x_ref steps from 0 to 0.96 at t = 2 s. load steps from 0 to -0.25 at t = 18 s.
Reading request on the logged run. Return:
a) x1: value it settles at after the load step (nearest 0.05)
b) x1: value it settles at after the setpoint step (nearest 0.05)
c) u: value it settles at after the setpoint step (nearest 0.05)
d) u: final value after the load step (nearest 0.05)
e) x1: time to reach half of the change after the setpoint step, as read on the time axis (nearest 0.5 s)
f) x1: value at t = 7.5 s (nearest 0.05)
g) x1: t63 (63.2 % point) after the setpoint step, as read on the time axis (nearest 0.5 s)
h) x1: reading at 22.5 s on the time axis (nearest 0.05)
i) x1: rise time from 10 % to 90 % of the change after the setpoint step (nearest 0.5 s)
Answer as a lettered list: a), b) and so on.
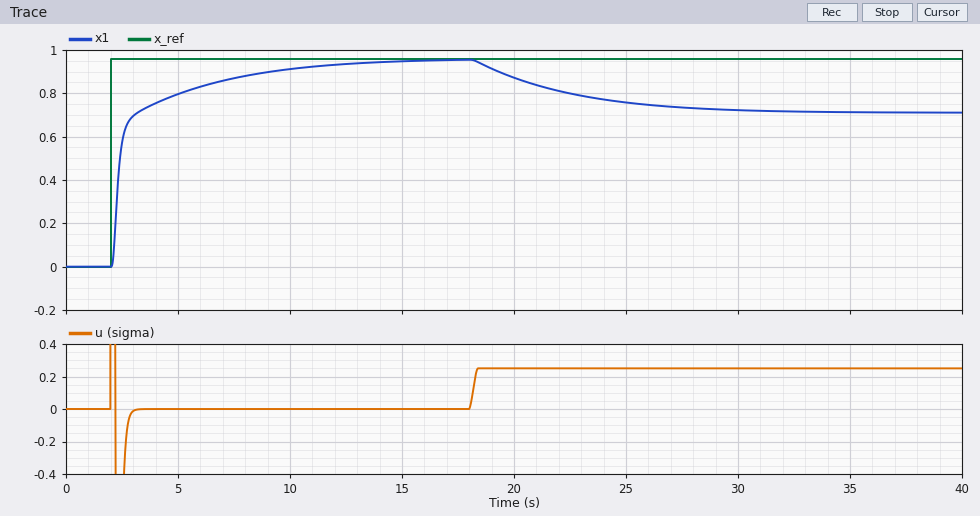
a) 0.70
b) 0.95
c) 0.00
d) 0.25
e) 2.5 s
f) 0.85
g) 2.5 s
h) 0.80
i) 5.0 s
